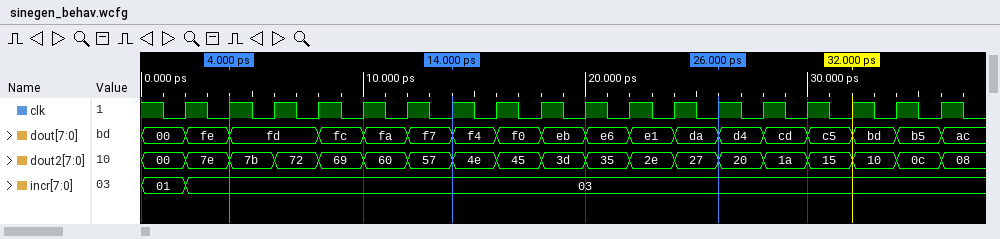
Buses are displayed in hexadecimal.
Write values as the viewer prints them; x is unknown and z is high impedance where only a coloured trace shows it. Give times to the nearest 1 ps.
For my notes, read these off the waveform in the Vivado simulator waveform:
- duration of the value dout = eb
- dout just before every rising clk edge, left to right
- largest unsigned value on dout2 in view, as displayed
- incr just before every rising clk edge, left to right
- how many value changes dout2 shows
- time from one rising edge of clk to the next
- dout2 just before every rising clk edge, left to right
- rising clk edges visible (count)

2 ps
00, fe, fd, fd, fc, fa, f7, f4, f0, eb, e6, e1, da, d4, cd, c5, bd, b5
7e
01, 03, 03, 03, 03, 03, 03, 03, 03, 03, 03, 03, 03, 03, 03, 03, 03, 03
18
2 ps
00, 7e, 7b, 72, 69, 60, 57, 4e, 45, 3d, 35, 2e, 27, 20, 1a, 15, 10, 0c
18
